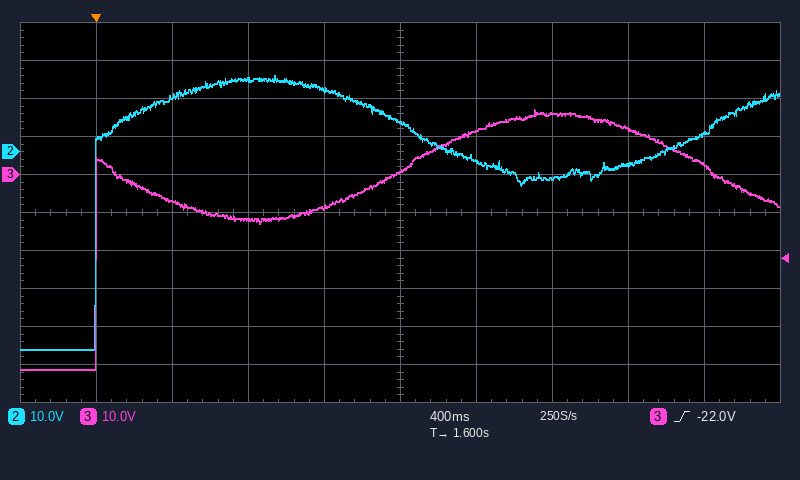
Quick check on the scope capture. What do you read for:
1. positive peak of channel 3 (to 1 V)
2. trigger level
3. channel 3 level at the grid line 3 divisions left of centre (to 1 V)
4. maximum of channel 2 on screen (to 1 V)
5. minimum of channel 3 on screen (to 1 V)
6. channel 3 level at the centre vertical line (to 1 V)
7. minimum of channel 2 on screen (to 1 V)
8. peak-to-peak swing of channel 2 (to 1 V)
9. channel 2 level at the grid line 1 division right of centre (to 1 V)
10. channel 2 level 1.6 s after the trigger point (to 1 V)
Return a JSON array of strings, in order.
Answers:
["17 V", "-22.0 V", "-7 V", "20 V", "-51 V", "1 V", "-52 V", "72 V", "-3 V", "8 V"]
